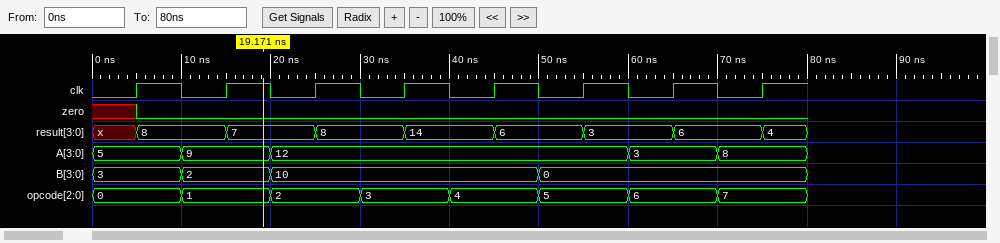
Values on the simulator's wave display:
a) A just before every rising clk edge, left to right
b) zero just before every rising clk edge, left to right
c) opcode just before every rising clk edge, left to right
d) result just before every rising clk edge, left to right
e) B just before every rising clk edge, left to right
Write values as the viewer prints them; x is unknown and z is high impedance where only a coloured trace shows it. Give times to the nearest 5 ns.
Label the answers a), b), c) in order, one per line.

a) 5, 9, 12, 12, 12, 12, 3, 8
b) x 0 0 0 0 0 0 0
c) 0, 1, 2, 3, 4, 5, 6, 7
d) x, 8, 7, 8, 14, 6, 3, 6
e) 3, 2, 10, 10, 10, 0, 0, 0
